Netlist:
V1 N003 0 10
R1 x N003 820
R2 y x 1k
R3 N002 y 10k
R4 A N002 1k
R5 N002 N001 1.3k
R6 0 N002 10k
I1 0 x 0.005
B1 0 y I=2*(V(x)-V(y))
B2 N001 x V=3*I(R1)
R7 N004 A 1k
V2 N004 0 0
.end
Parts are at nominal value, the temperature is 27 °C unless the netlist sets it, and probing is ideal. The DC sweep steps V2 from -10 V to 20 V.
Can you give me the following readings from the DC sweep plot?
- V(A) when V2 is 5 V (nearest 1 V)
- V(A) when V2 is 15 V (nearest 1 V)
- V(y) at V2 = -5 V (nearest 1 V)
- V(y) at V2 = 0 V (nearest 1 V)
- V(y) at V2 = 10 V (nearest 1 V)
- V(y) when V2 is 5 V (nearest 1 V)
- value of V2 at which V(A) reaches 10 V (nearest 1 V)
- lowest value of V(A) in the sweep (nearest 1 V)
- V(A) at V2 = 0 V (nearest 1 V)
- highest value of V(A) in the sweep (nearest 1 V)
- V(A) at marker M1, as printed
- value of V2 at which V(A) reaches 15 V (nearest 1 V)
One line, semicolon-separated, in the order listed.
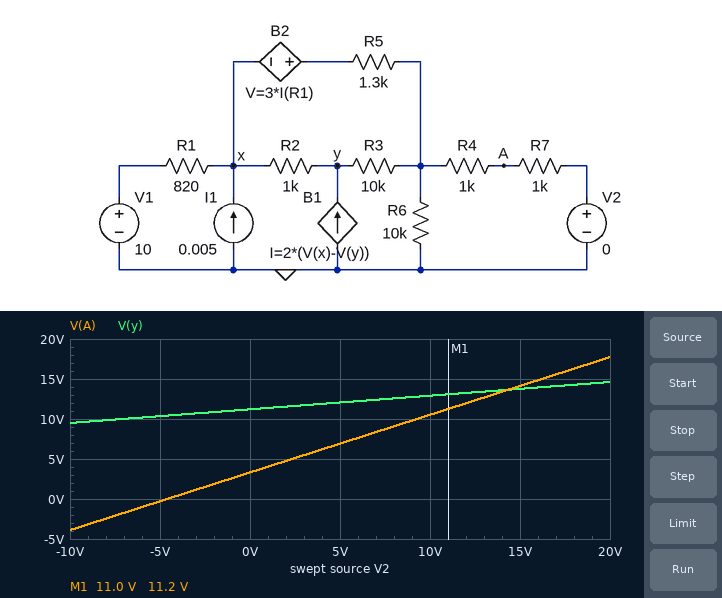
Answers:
7 V; 14 V; 10 V; 11 V; 13 V; 12 V; 9 V; -4 V; 3 V; 18 V; 11.2 V; 16 V
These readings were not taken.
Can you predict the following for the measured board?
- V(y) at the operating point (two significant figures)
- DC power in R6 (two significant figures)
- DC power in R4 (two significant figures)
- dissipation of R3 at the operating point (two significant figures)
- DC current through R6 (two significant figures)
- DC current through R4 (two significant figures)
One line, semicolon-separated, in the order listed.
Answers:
11 V; 4.4 mW; 11 mW; 2.1 mW; 660 µA; 3.3 mA
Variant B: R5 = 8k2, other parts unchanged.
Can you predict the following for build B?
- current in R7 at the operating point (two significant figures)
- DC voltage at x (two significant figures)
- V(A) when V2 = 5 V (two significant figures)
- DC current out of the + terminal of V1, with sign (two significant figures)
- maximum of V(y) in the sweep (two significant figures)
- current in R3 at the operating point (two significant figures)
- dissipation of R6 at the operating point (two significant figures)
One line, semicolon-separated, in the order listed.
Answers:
1.8 mA; 13 V; 5.8 V; -3.8 mA; 14 V; 960 µA; 1.3 mW
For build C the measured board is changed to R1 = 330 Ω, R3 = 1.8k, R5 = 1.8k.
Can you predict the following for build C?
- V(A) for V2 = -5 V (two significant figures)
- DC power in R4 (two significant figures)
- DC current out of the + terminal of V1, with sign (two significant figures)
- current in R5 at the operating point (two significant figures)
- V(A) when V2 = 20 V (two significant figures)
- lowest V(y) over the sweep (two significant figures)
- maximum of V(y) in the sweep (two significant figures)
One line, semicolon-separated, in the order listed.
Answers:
240 mV; 13 mW; -2.9 mA; 2.1 mA; 17 V; 10 V; 12 V
